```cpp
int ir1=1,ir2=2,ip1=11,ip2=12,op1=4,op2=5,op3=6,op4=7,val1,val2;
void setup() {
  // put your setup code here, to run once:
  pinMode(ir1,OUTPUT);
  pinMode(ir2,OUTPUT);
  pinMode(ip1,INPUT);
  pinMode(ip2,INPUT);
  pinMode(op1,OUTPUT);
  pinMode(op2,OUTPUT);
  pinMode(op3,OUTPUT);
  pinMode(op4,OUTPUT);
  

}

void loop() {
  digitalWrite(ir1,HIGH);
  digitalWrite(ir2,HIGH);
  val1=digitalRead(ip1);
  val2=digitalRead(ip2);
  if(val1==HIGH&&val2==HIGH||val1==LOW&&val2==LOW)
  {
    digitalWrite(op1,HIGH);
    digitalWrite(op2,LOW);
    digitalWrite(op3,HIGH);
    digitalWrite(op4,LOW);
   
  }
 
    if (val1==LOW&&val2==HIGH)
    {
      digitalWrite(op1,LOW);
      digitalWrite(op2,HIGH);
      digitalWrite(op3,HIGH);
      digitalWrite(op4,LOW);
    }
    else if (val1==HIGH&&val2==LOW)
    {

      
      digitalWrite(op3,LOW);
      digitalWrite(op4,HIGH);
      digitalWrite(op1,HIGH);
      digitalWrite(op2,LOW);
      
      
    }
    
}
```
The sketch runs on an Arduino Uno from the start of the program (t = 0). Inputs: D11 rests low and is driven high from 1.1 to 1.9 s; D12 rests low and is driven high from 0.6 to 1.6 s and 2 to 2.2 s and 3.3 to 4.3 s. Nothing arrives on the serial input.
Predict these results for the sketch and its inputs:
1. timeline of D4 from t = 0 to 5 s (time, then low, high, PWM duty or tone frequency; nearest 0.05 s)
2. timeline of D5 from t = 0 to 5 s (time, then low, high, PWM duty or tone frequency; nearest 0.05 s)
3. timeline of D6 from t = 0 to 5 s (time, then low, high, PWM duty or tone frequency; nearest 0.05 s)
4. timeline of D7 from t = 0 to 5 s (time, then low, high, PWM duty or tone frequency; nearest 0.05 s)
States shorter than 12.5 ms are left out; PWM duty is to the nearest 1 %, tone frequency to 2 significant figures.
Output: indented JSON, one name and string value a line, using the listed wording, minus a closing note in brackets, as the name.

{
  "timeline of D4 from t = 0 to 5 s": "0 s high; 0.6 s low; 1.1 s high; 2 s low; 2.2 s high; 3.3 s low; 4.3 s high",
  "timeline of D5 from t = 0 to 5 s": "0 s low; 0.6 s high; 1.1 s low; 2 s high; 2.2 s low; 3.3 s high; 4.3 s low",
  "timeline of D6 from t = 0 to 5 s": "0 s high; 1.6 s low; 1.9 s high",
  "timeline of D7 from t = 0 to 5 s": "0 s low; 1.6 s high; 1.9 s low"
}
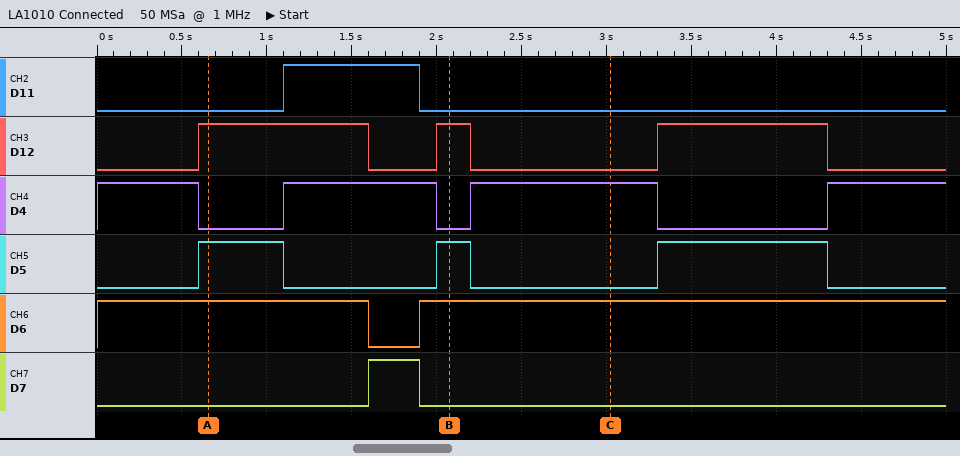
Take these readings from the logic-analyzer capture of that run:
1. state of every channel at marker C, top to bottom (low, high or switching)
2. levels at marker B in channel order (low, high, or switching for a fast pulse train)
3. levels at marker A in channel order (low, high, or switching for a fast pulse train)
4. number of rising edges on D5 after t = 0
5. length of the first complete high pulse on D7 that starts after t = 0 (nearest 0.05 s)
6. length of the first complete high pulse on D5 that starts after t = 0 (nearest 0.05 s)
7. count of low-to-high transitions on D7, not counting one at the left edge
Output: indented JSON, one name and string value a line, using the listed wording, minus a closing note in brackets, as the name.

{
  "state of every channel at marker C, top to bottom": "D11 low, D12 low, D4 high, D5 low, D6 high, D7 low",
  "levels at marker B in channel order": "D11 low, D12 high, D4 low, D5 high, D6 high, D7 low",
  "levels at marker A in channel order": "D11 low, D12 high, D4 low, D5 high, D6 high, D7 low",
  "number of rising edges on D5 after t = 0": "3",
  "length of the first complete high pulse on D7 that starts after t = 0": "0.30 s",
  "length of the first complete high pulse on D5 that starts after t = 0": "0.50 s",
  "count of low-to-high transitions on D7, not counting one at the left edge": "1"
}
